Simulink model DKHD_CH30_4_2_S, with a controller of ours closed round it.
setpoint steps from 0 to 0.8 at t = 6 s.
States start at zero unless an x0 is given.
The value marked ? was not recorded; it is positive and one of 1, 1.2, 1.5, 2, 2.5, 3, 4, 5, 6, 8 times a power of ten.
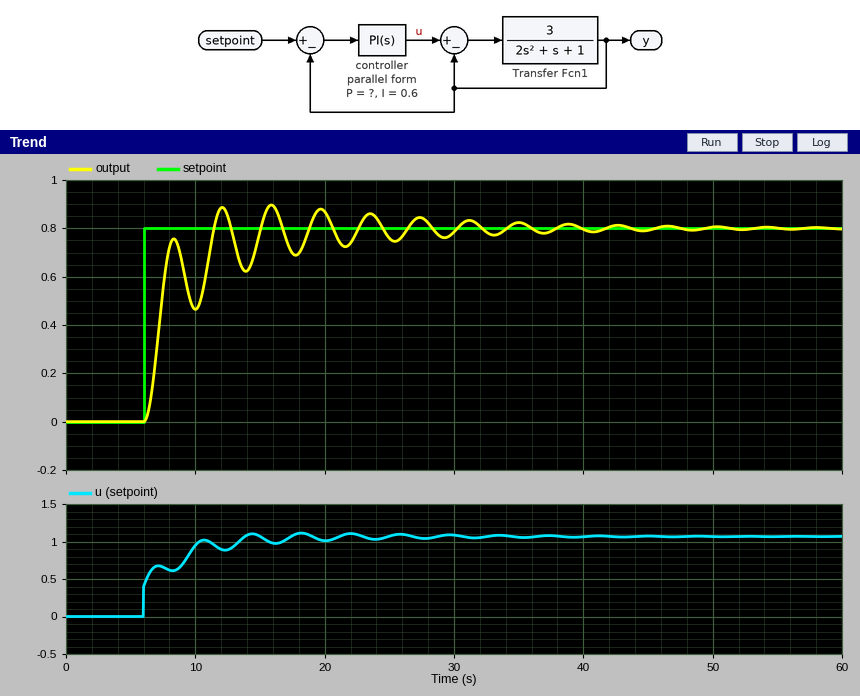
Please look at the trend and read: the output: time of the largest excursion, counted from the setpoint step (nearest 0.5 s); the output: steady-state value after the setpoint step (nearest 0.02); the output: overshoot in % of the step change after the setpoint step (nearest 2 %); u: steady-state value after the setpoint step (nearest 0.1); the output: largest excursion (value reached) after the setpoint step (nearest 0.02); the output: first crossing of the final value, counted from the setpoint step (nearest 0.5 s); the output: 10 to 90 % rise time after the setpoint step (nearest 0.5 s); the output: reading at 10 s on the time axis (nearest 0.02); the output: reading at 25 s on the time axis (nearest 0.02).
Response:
10.0 s
0.80
12 %
1.1
0.90
5.5 s
1.5 s
0.46
0.76
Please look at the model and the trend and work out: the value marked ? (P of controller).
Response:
0.5
